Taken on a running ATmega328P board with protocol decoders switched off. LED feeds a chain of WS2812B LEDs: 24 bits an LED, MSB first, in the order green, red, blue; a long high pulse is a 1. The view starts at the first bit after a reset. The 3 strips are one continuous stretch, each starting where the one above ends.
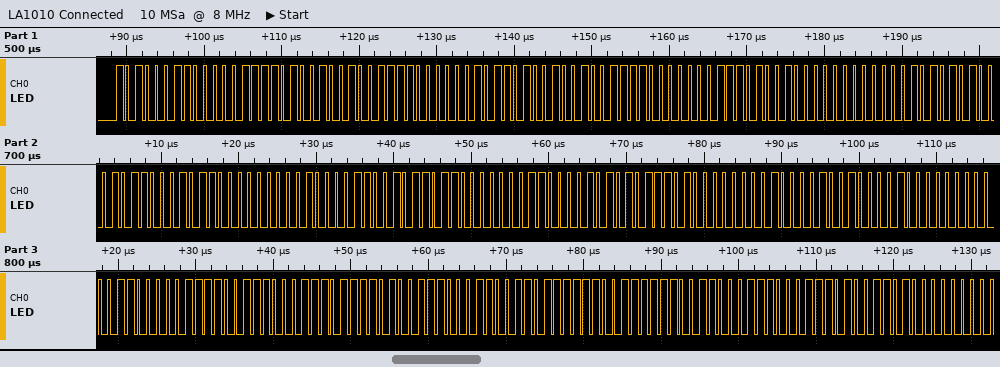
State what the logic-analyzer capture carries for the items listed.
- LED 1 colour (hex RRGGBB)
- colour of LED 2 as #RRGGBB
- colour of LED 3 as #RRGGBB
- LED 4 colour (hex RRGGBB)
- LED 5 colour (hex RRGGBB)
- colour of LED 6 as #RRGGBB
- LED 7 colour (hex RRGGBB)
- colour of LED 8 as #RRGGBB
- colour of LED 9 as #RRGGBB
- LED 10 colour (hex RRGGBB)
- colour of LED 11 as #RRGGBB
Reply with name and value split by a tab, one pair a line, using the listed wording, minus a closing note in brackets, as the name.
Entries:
LED 1 colour	#07A3A4
colour of LED 2 as #RRGGBB	#059EA4
colour of LED 3 as #RRGGBB	#039EA4
LED 4 colour	#2A008B
LED 5 colour	#001686
colour of LED 6 as #RRGGBB	#015B85
LED 7 colour	#005D84
colour of LED 8 as #RRGGBB	#008460
colour of LED 9 as #RRGGBB	#8EF3F4
LED 10 colour	#37E3E7
colour of LED 11 as #RRGGBB	#38E6E9
